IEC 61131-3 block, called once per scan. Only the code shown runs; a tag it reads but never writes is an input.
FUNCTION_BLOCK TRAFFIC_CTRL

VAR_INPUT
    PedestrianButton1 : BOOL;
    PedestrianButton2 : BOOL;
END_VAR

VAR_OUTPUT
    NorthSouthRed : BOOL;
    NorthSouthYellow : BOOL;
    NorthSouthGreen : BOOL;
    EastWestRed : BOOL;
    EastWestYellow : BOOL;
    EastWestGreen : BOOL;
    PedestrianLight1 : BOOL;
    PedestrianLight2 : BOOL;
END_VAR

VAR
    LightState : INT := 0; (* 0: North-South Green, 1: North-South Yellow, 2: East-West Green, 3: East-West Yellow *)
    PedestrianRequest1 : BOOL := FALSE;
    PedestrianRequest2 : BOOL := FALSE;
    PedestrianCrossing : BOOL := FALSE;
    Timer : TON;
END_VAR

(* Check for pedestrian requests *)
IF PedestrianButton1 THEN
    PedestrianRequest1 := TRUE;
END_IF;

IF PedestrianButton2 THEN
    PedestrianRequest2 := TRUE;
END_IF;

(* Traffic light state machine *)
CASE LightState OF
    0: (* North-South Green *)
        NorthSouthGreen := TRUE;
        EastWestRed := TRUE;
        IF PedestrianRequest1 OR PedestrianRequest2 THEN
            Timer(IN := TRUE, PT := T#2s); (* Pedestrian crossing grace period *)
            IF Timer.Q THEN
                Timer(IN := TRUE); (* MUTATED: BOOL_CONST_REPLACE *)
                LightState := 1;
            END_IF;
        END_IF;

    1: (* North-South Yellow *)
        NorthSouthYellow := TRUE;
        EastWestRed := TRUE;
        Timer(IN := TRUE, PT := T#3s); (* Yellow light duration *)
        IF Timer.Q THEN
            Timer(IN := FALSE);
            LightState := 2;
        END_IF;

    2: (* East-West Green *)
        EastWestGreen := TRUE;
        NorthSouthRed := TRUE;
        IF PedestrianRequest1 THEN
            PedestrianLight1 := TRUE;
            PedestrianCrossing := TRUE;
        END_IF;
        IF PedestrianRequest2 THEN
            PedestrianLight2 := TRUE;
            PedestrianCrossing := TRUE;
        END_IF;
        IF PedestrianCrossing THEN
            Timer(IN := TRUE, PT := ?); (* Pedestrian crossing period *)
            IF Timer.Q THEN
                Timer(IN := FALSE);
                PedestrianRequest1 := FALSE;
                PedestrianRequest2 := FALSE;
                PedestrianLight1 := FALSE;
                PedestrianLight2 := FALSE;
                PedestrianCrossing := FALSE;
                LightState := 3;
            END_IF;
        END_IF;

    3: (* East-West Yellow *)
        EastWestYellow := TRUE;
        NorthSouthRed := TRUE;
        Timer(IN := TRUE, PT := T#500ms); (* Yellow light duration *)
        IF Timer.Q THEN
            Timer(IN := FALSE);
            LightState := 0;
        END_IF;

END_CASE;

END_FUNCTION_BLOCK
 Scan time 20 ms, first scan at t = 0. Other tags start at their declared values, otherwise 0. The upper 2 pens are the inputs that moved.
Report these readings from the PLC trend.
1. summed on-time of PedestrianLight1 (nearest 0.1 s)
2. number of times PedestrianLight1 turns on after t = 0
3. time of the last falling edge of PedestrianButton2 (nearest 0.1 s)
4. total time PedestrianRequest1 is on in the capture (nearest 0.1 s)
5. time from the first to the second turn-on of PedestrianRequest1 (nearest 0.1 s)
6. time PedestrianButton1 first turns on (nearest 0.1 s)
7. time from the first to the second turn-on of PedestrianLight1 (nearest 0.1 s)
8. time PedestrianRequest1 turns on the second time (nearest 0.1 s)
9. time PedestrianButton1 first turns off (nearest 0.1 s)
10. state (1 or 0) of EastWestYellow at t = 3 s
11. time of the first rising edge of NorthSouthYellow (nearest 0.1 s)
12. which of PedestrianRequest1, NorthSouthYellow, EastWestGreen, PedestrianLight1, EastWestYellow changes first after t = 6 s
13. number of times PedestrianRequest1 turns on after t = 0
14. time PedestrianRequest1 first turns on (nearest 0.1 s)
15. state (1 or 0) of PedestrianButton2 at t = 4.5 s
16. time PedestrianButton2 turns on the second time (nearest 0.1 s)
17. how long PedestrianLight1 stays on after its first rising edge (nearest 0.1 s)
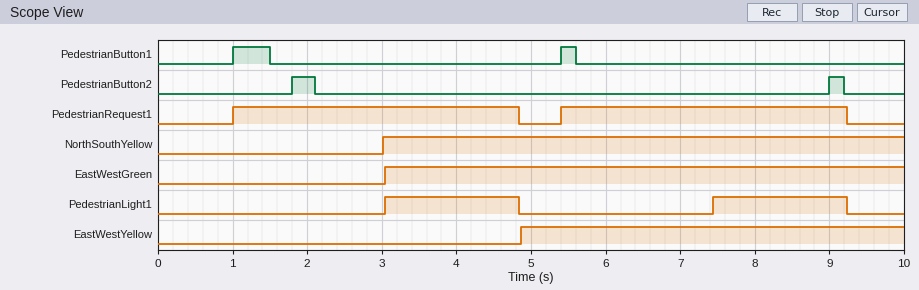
3.6 s
2
9.2 s
7.7 s
4.4 s
1.0 s
4.4 s
5.4 s
1.5 s
0
3.0 s
PedestrianLight1
2
1.0 s
0
9.0 s
1.8 s
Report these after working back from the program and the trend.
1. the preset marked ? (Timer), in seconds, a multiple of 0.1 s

1.8 s
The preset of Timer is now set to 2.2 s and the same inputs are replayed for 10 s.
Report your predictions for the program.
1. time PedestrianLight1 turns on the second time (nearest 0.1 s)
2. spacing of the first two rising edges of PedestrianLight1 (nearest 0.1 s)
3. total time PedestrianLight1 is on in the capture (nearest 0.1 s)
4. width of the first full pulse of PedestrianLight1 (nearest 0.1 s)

7.8 s
4.8 s
4.4 s
2.2 s
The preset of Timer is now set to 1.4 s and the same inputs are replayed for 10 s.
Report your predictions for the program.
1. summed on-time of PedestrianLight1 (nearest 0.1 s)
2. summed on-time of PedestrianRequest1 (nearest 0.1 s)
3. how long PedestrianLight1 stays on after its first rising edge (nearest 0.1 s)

2.8 s
6.9 s
1.4 s
